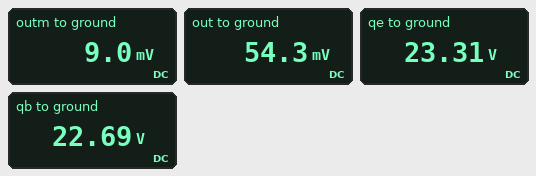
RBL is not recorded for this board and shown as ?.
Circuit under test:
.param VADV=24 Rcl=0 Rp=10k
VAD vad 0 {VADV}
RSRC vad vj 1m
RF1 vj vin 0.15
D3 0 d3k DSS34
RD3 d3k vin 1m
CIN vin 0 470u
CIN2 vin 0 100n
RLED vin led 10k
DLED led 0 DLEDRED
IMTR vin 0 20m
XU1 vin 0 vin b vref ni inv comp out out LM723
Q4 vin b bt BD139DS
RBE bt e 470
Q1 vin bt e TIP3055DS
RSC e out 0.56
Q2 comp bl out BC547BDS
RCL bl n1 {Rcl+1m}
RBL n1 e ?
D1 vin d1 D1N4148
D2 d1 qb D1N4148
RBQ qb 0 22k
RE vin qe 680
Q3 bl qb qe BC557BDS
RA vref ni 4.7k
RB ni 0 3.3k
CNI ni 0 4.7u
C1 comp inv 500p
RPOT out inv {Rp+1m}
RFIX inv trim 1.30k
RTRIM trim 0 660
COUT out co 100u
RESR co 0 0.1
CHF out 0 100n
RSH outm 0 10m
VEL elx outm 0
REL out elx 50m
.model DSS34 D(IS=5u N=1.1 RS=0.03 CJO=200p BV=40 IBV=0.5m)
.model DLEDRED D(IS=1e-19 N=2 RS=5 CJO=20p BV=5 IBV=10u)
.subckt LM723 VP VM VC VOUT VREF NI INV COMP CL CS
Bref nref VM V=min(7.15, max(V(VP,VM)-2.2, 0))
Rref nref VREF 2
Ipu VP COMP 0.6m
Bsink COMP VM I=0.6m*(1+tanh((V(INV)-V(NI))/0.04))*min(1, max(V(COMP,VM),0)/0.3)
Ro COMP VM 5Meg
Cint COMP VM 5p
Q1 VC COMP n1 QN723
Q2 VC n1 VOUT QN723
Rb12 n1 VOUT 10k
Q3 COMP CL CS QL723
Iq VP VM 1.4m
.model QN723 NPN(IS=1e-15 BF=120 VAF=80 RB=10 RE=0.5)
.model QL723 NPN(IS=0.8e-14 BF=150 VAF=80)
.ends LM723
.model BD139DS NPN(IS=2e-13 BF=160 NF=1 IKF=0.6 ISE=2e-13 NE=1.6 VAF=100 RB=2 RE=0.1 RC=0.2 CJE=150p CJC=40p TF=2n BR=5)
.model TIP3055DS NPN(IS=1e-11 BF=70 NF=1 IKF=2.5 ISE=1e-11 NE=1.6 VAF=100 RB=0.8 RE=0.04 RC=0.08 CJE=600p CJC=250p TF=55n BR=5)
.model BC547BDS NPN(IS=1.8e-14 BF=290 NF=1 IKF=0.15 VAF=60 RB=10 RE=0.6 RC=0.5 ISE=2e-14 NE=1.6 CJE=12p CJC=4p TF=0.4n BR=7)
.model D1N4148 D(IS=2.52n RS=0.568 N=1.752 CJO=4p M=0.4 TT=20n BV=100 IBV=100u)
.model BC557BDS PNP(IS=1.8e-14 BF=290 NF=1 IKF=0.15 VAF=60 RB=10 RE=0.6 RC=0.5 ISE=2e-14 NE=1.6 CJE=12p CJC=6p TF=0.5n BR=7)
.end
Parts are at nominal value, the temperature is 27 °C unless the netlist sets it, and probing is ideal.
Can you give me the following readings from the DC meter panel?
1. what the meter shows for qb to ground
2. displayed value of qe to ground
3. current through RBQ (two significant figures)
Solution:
22.69 V
23.31 V
1.0 mA
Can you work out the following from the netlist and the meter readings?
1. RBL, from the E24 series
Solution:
150 Ω
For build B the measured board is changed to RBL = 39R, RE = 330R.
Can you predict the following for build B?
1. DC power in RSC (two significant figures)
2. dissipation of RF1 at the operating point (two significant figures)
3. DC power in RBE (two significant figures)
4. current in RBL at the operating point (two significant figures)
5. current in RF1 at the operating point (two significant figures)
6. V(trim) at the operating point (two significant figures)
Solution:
570 mW
160 mW
1.1 mW
1.6 mA
1.0 A
3.3 mV
